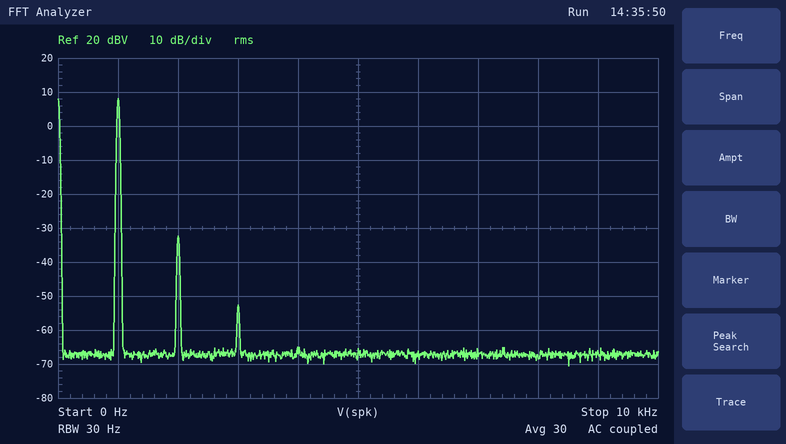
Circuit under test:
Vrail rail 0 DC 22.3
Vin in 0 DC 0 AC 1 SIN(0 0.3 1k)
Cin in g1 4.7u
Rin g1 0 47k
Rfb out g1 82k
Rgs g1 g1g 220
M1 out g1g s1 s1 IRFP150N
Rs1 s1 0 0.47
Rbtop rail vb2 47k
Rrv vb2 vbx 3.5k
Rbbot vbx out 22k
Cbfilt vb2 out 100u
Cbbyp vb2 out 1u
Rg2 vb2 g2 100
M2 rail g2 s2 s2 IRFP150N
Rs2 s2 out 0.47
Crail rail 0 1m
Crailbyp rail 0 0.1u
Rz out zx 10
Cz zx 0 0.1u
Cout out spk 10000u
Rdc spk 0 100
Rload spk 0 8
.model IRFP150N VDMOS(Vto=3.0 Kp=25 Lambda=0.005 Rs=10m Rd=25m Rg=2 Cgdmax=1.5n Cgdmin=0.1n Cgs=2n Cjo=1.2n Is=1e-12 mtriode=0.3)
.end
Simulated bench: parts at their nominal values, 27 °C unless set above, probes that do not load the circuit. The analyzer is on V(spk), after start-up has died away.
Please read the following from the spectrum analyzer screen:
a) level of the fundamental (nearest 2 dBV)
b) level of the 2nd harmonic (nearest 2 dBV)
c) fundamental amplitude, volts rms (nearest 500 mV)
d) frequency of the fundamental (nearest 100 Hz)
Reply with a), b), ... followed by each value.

a) 8 dBV
b) -32 dBV
c) 2.5 V
d) 1.0 kHz
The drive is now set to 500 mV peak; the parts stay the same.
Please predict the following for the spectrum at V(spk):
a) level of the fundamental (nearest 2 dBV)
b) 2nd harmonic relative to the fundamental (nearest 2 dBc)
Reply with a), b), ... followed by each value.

a) 12 dBV
b) -36 dBc
